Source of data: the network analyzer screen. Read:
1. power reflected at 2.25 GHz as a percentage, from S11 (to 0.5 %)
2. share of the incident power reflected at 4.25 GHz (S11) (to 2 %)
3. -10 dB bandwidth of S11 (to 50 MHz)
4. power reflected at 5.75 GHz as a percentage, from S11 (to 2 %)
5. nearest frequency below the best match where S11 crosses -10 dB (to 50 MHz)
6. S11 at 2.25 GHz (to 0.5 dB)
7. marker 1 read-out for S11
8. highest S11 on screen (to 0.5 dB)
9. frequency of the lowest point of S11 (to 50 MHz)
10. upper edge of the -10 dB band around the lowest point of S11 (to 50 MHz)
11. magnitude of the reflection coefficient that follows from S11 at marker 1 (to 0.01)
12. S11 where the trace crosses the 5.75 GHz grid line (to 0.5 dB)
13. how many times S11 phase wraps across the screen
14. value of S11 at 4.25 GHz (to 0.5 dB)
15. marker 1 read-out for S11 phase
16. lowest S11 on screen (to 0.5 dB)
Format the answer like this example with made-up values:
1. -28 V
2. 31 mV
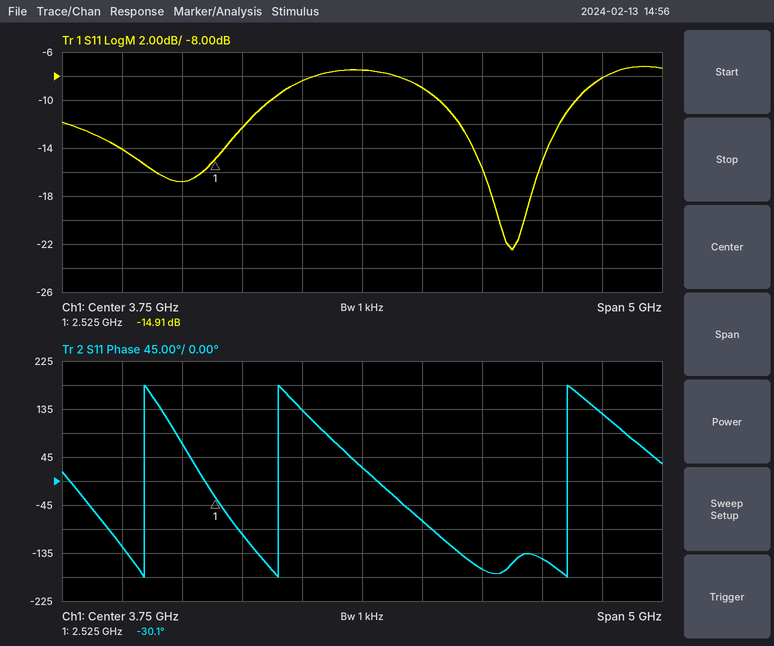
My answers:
1. 2.0 %
2. 12 %
3. 1.15 GHz
4. 16 %
5. 4.40 GHz
6. -17.0 dB
7. -14.91 dB
8. -7.0 dB
9. 5.00 GHz
10. 5.55 GHz
11. 0.18
12. -8.0 dB
13. 3
14. -9.0 dB
15. -30.1°
16. -22.5 dB
